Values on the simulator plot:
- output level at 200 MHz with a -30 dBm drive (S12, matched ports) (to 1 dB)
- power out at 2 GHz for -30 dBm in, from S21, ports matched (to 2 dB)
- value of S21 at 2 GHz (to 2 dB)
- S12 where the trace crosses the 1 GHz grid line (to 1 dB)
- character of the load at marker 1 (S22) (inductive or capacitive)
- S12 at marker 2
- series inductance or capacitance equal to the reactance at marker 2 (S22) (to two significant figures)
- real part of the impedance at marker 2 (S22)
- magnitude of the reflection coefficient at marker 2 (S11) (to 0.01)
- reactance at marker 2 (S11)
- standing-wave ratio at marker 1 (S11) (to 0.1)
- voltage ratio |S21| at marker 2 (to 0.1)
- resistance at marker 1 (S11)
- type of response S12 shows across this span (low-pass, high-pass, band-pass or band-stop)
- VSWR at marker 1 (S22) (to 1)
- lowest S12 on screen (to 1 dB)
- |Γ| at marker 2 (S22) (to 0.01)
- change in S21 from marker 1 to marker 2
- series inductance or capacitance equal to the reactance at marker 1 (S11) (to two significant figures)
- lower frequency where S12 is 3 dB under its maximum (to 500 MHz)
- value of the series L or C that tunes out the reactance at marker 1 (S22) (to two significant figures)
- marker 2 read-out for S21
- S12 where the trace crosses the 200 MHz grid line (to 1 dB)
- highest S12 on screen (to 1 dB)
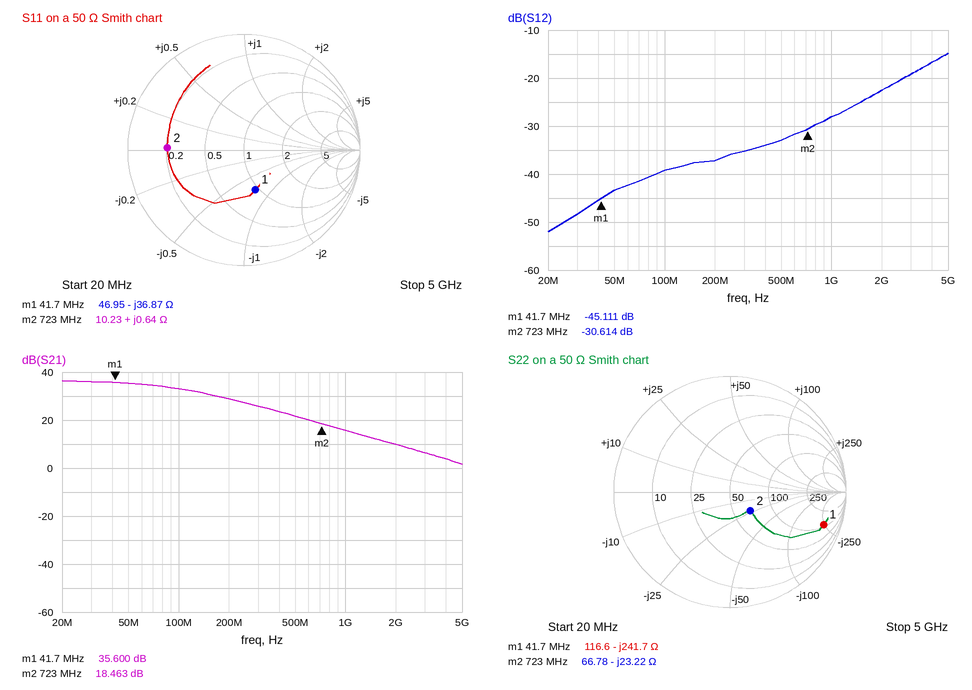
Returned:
-67 dBm
-20 dBm
10 dB
-28 dB
capacitive
-30.614 dB
9.5 pF
66.78 Ω
0.66
+0.64 Ω
2.1
8.4
46.95 Ω
high-pass
13
-52 dB
0.24
-17.137 dB
100 pF
3.5 GHz
920 nH
18.463 dB
-37 dB
-15 dB
